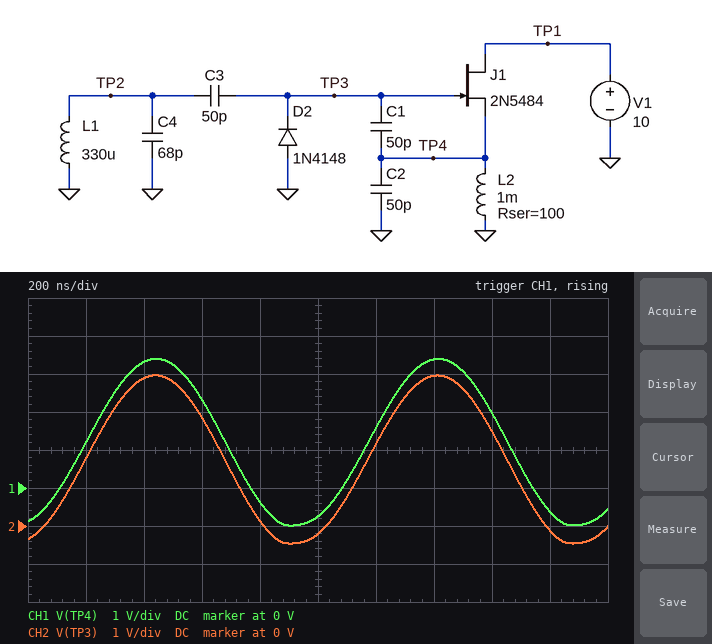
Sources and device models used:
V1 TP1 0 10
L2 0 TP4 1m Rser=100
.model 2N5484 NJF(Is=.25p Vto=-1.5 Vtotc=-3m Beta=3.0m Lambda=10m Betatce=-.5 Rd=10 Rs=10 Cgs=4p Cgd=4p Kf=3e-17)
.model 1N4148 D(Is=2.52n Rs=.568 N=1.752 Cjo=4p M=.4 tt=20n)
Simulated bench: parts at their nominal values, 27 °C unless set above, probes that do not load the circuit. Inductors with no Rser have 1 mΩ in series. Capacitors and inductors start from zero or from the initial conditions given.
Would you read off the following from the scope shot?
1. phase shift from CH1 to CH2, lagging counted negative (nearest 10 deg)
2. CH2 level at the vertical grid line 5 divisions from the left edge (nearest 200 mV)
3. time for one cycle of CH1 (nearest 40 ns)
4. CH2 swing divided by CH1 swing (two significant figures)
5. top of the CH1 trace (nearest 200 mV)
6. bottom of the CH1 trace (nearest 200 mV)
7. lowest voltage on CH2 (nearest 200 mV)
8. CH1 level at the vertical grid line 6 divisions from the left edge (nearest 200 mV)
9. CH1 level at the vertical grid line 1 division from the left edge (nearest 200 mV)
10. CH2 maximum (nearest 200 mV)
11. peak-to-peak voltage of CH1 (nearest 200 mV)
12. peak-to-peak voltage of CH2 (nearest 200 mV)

0 deg
-200 mV
960 ns
1.0
3.4 V
-1.0 V
-400 mV
1.6 V
1.2 V
4.0 V
4.4 V
4.4 V
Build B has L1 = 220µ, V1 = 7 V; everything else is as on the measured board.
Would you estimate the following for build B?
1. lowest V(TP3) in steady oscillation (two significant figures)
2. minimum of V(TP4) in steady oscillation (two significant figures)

-490 mV
-1.0 V
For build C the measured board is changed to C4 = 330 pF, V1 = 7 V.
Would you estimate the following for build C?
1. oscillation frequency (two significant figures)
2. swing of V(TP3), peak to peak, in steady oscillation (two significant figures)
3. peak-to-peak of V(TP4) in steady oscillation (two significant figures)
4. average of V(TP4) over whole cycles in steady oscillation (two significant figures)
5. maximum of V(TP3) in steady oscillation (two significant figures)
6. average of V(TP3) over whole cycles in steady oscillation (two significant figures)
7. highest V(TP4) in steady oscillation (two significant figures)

480 kHz
300 mV
290 mV
540 mV
550 mV
400 mV
690 mV
